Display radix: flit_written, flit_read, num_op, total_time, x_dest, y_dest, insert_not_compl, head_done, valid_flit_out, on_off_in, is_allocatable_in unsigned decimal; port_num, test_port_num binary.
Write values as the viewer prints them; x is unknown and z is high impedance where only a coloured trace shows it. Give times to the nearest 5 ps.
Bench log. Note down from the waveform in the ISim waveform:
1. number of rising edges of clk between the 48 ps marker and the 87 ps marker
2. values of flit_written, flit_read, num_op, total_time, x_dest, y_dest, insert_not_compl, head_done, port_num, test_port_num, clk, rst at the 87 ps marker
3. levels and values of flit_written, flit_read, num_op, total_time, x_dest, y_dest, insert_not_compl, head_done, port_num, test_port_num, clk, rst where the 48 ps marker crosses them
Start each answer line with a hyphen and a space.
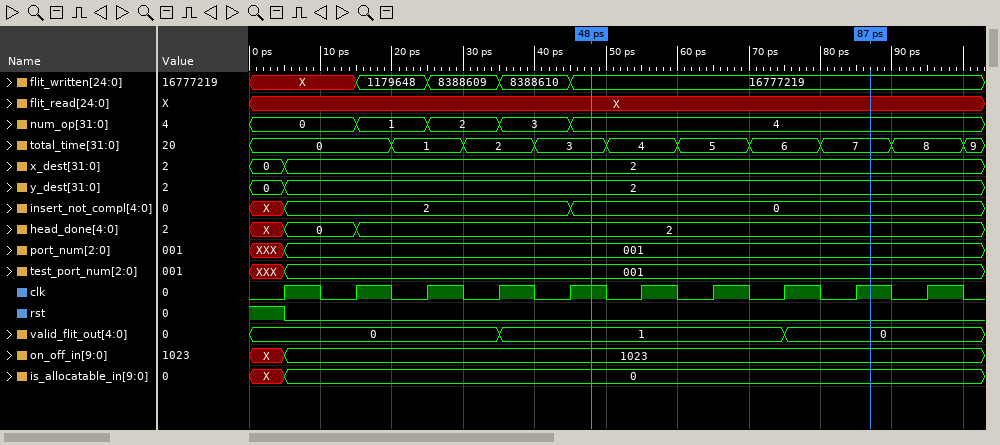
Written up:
- 4
- flit_written=16777219, flit_read=X, num_op=4, total_time=7, x_dest=2, y_dest=2, insert_not_compl=0, head_done=2, port_num=001, test_port_num=001, clk=1, rst=0
- flit_written=16777219, flit_read=X, num_op=4, total_time=3, x_dest=2, y_dest=2, insert_not_compl=0, head_done=2, port_num=001, test_port_num=001, clk=1, rst=0
